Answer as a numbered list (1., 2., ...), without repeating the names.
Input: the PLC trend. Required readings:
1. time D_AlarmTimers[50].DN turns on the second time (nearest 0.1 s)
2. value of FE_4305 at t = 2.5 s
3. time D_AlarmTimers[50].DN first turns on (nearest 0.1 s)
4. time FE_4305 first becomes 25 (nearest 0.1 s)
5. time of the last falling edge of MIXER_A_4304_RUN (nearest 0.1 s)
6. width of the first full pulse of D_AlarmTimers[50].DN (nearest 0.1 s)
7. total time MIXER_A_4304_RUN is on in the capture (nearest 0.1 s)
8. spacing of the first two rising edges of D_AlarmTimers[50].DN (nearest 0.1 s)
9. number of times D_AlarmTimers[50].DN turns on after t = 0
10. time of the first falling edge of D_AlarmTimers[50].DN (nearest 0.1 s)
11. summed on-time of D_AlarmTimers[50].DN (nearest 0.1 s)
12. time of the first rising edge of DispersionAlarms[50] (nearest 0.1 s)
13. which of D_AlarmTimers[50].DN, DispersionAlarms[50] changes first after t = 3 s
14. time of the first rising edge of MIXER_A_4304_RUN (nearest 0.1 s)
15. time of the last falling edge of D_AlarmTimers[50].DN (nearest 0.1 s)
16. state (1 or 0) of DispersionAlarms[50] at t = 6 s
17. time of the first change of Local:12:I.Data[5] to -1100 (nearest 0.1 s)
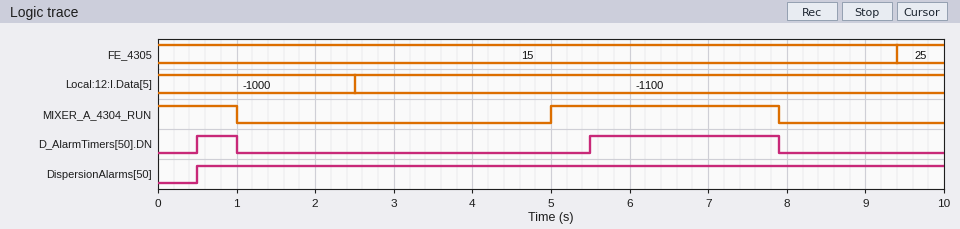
1. 5.5 s
2. 15
3. 0.5 s
4. 9.4 s
5. 7.9 s
6. 0.5 s
7. 3.9 s
8. 5.0 s
9. 2
10. 1.0 s
11. 2.9 s
12. 0.5 s
13. D_AlarmTimers[50].DN
14. 5.0 s
15. 7.9 s
16. 1
17. 2.5 s
